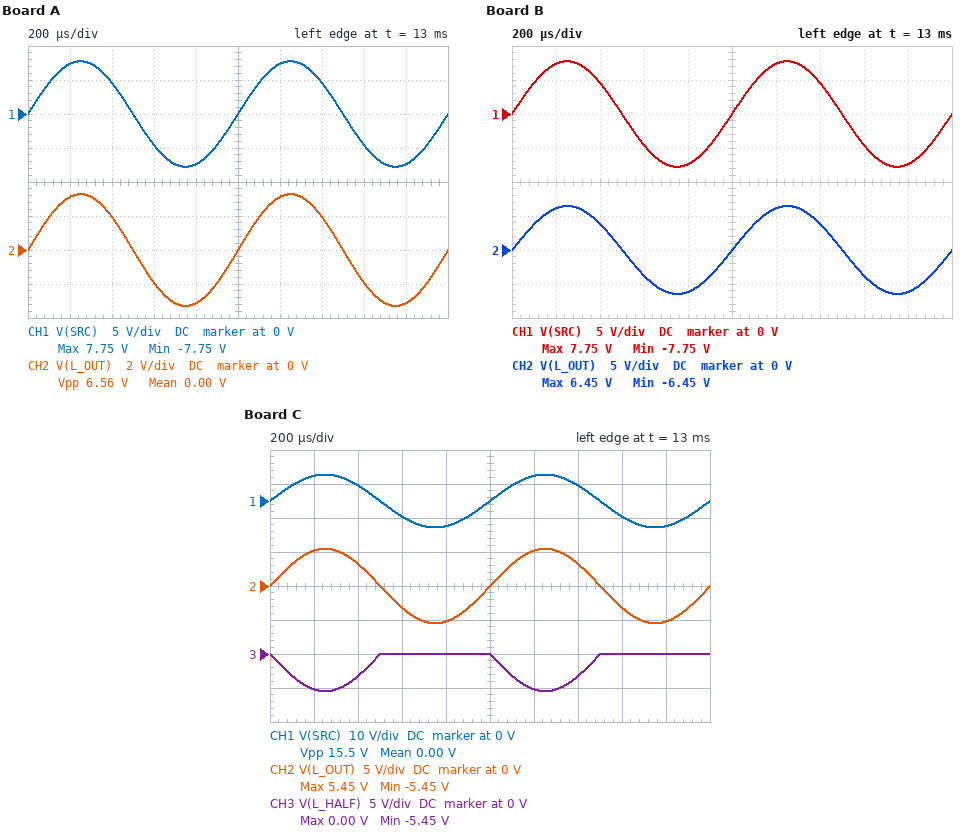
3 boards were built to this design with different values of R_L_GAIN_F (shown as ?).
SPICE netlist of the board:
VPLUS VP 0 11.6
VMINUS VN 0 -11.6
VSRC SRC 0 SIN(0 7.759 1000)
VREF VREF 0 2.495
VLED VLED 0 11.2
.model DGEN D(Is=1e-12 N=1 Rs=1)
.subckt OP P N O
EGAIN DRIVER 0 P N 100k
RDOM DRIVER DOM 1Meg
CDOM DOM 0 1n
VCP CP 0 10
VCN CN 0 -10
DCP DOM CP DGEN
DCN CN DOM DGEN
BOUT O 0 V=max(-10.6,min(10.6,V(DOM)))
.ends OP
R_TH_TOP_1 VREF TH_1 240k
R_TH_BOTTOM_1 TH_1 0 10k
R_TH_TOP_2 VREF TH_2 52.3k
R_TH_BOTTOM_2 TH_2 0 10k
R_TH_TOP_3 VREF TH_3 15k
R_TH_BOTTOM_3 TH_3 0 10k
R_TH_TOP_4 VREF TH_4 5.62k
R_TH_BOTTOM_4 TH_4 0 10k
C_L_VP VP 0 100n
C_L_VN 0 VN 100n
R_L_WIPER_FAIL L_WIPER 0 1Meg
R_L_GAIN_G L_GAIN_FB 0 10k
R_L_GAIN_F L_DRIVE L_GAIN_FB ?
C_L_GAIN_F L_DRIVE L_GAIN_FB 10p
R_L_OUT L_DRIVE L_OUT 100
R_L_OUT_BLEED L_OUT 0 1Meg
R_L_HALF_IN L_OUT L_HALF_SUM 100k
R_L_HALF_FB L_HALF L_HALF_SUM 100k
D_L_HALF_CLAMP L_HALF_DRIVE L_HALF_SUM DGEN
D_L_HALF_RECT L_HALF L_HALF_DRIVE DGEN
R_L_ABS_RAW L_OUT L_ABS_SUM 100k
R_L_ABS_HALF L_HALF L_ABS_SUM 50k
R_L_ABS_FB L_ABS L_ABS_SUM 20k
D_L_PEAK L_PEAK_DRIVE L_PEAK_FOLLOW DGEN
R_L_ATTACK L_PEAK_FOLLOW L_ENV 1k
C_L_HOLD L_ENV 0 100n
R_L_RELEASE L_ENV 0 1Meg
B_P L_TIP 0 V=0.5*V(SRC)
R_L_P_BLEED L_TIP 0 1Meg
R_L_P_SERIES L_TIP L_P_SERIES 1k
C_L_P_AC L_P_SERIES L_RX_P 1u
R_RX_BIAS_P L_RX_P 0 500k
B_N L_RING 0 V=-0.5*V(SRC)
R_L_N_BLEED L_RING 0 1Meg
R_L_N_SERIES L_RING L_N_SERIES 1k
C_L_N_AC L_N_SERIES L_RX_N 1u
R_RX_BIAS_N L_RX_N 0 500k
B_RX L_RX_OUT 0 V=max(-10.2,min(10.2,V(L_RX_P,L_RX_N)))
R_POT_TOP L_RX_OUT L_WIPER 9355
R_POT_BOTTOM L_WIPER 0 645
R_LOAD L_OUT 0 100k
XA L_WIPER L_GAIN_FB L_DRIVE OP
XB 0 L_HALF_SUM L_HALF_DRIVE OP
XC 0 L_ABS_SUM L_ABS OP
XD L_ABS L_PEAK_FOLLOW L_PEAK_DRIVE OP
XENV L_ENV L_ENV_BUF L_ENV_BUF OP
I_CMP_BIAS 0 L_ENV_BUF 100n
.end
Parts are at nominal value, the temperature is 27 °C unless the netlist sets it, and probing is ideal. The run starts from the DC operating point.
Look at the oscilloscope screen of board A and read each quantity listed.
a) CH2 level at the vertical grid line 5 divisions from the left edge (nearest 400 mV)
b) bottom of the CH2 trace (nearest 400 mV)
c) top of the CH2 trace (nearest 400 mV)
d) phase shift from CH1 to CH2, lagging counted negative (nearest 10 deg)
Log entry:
0 V
-3.2 V
3.2 V
0 deg
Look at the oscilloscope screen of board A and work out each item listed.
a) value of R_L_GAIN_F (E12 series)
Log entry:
56 kΩ
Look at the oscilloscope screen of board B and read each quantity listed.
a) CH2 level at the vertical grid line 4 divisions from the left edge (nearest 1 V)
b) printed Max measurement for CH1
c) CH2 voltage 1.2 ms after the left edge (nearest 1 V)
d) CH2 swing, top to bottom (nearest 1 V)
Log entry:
-6 V
7.75 V
6 V
13 V
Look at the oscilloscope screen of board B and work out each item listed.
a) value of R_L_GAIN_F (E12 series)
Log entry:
120 kΩ
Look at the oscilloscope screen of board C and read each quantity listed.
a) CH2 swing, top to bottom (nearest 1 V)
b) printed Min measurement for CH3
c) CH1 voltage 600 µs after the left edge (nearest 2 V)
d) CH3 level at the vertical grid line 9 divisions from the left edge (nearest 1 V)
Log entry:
11 V
-5.45 V
-4 V
0 V
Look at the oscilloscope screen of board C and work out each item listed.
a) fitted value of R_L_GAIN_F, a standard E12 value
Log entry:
100 kΩ
